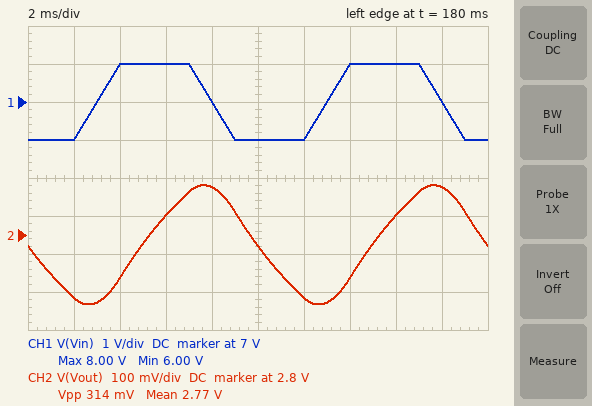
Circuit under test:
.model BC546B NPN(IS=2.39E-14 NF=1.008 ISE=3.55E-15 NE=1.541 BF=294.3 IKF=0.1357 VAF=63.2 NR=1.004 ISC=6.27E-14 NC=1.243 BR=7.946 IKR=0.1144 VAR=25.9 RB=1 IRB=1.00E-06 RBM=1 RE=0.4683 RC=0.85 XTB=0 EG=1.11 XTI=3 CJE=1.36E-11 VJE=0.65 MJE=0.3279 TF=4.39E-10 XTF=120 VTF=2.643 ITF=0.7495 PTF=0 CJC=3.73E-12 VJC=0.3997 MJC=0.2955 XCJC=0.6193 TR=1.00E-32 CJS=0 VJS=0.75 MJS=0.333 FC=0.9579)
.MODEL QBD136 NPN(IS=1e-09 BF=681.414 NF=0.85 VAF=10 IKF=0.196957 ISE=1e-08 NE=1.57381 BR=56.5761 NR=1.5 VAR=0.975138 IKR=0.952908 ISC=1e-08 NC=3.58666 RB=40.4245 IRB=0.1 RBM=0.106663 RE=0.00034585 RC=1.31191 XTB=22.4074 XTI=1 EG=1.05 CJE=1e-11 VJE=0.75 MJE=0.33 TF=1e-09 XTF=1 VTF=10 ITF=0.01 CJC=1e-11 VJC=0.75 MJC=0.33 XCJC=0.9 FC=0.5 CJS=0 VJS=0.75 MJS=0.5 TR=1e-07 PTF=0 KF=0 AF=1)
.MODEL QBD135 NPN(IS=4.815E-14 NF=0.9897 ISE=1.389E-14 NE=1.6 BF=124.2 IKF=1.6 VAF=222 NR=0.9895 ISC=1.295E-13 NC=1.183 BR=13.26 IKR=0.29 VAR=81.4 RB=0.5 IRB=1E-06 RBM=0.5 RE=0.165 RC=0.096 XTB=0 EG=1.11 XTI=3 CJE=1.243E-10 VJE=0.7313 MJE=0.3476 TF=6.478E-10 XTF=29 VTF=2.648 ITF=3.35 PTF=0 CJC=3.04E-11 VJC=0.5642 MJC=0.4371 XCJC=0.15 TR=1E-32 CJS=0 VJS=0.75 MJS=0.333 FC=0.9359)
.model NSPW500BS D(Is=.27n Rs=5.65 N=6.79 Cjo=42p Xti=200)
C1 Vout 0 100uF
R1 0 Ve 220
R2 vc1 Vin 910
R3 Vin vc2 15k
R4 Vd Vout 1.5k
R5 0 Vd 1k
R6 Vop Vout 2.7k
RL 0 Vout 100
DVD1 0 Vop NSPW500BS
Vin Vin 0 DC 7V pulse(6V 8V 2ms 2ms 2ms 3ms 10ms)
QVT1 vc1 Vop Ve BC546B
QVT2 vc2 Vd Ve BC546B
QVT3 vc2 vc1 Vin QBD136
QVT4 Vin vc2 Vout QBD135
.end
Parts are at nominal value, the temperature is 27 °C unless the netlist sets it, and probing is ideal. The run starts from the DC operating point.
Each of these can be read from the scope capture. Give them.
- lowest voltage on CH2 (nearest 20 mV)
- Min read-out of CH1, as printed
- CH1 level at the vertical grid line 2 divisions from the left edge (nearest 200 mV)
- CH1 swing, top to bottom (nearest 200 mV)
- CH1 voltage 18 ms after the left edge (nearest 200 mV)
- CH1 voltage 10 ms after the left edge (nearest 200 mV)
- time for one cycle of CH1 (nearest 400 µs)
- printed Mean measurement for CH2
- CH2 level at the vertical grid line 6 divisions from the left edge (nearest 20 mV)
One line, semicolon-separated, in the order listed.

2.62 V; 6.00 V; 8.0 V; 2.0 V; 7.0 V; 6.0 V; 10.0 ms; 2.77 V; 2.64 V
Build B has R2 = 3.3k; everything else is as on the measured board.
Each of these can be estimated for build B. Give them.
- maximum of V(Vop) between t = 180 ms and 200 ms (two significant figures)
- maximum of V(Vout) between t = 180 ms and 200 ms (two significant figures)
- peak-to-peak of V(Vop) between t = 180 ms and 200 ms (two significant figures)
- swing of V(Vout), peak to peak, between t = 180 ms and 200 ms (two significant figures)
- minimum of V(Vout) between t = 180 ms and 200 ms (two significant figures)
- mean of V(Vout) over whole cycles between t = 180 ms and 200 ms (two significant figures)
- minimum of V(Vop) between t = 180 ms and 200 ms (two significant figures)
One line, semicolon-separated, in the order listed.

1.3 V; 2.8 V; 150 mV; 380 mV; 2.5 V; 2.6 V; 1.2 V
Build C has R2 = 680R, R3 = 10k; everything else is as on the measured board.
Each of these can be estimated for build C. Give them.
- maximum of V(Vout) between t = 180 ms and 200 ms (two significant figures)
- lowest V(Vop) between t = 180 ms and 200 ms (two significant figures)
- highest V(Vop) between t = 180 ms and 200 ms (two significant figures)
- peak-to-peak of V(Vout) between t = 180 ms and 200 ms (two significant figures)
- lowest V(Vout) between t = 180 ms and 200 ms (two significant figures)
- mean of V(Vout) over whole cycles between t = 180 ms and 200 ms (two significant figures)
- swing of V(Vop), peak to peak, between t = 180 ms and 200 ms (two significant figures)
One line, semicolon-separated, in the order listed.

3.6 V; 2.2 V; 2.7 V; 450 mV; 3.2 V; 3.4 V; 490 mV
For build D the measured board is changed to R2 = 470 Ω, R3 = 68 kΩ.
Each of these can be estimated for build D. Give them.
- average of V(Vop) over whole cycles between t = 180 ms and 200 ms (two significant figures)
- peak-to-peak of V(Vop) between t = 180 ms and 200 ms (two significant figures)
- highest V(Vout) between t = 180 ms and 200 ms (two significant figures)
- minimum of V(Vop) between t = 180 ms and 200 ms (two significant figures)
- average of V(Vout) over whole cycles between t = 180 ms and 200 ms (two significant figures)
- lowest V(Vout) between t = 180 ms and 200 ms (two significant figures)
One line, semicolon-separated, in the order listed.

2.4 V; 640 mV; 2.7 V; 2.0 V; 2.5 V; 2.1 V
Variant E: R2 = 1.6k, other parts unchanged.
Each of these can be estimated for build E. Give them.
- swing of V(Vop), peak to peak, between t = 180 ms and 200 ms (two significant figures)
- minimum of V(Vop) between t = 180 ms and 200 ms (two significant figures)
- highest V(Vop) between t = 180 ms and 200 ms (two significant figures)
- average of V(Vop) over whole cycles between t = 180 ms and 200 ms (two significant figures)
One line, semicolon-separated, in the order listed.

250 mV; 1.5 V; 1.7 V; 1.6 V
